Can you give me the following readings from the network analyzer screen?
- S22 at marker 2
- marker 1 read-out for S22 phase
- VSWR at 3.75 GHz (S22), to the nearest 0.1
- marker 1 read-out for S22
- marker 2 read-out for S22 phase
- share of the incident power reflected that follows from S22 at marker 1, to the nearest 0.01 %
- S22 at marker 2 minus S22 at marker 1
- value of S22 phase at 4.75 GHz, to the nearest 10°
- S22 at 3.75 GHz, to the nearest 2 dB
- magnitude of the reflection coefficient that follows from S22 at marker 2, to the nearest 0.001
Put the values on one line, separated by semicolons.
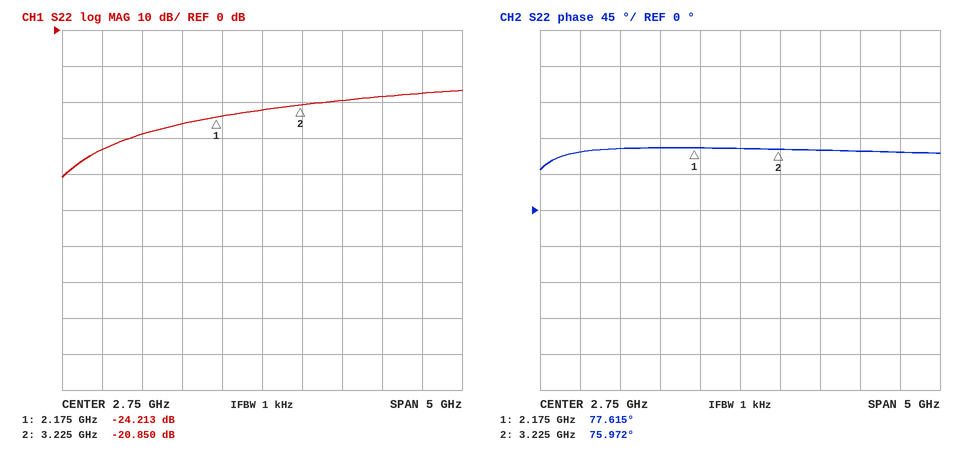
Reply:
-20.850 dB; 77.615°; 1.2; -24.213 dB; 75.972°; 0.38 %; 3.363 dB; 70°; -20 dB; 0.091
